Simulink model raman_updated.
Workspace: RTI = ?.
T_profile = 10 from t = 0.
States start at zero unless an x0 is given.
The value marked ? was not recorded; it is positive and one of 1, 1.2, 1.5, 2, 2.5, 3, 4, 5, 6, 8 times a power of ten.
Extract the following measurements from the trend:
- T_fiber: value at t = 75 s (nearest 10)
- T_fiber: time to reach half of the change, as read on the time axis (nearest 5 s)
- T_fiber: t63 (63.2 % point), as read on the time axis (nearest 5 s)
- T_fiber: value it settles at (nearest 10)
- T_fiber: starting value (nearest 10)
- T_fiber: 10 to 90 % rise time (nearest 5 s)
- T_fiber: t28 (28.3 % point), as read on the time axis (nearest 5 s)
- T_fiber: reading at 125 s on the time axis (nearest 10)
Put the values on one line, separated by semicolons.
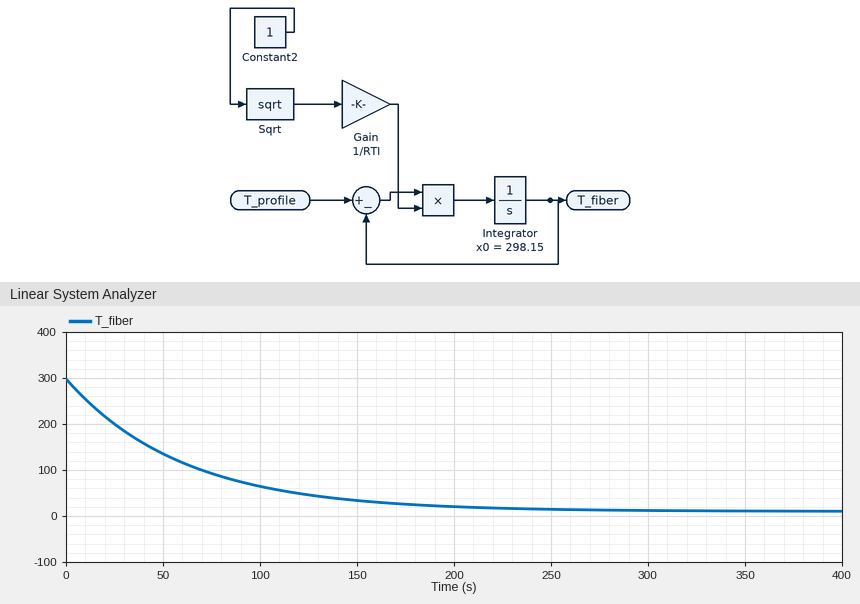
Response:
90; 40 s; 60 s; 10; 300; 130 s; 20 s; 50
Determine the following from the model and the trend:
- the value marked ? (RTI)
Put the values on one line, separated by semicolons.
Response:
60
